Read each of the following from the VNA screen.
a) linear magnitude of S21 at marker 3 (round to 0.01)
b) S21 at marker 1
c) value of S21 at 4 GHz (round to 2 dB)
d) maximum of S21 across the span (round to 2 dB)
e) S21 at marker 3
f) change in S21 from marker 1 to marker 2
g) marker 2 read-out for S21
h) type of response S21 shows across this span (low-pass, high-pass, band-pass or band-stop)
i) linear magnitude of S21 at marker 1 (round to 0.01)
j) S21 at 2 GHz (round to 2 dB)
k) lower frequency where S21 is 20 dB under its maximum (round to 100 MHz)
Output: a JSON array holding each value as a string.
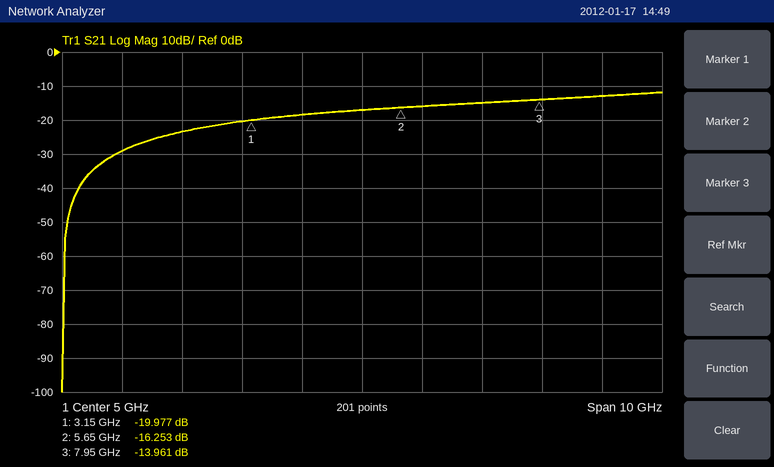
["0.20", "-19.977 dB", "-18 dB", "-12 dB", "-13.961 dB", "3.724 dB", "-16.253 dB", "high-pass", "0.10", "-24 dB", "700 MHz"]
